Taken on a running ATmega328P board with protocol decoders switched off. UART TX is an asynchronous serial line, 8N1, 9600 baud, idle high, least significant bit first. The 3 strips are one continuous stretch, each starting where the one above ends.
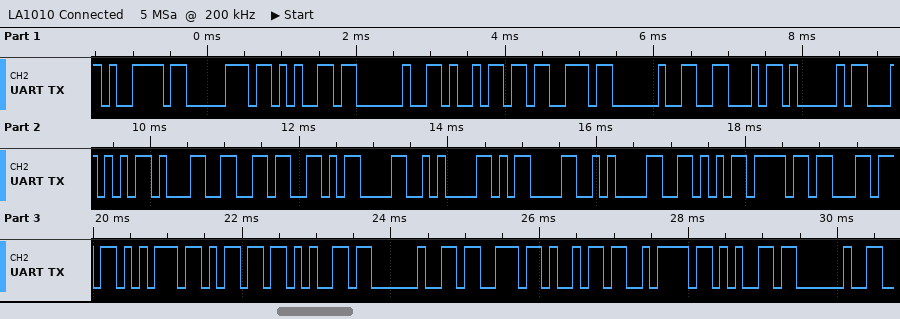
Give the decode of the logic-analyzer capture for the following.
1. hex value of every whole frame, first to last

79 70 65 20 69 73 20 46 41 54 31 36 0D 0A 0D 0A 56 6F 6C 75 6D 65 20 73 69 7A 65 20
